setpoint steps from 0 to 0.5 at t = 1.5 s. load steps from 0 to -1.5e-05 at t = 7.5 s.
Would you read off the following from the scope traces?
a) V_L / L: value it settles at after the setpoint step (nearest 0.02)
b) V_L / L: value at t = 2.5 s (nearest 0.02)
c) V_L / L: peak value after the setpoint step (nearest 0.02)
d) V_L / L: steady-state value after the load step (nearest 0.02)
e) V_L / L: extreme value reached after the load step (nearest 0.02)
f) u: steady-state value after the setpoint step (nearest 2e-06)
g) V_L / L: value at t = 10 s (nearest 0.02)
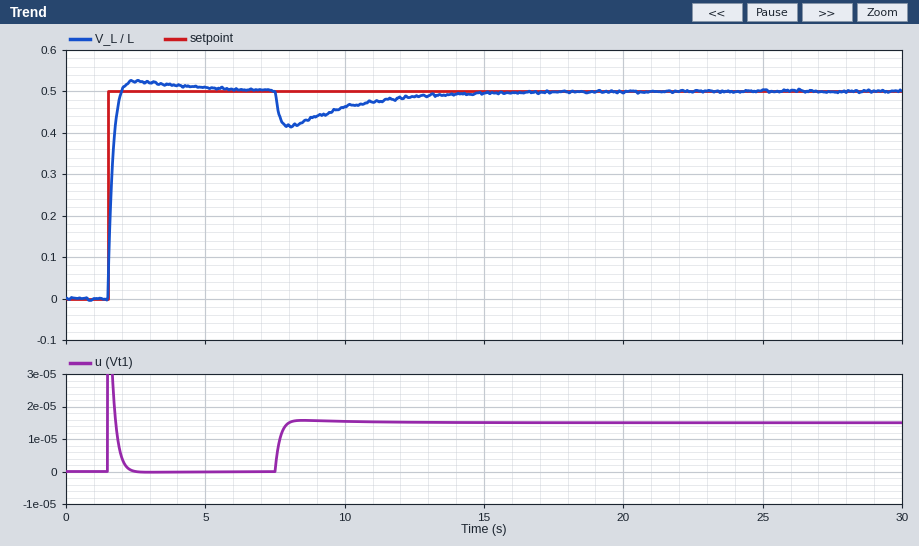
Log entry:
0.50
0.52
0.52
0.50
0.42
0.000000
0.46
